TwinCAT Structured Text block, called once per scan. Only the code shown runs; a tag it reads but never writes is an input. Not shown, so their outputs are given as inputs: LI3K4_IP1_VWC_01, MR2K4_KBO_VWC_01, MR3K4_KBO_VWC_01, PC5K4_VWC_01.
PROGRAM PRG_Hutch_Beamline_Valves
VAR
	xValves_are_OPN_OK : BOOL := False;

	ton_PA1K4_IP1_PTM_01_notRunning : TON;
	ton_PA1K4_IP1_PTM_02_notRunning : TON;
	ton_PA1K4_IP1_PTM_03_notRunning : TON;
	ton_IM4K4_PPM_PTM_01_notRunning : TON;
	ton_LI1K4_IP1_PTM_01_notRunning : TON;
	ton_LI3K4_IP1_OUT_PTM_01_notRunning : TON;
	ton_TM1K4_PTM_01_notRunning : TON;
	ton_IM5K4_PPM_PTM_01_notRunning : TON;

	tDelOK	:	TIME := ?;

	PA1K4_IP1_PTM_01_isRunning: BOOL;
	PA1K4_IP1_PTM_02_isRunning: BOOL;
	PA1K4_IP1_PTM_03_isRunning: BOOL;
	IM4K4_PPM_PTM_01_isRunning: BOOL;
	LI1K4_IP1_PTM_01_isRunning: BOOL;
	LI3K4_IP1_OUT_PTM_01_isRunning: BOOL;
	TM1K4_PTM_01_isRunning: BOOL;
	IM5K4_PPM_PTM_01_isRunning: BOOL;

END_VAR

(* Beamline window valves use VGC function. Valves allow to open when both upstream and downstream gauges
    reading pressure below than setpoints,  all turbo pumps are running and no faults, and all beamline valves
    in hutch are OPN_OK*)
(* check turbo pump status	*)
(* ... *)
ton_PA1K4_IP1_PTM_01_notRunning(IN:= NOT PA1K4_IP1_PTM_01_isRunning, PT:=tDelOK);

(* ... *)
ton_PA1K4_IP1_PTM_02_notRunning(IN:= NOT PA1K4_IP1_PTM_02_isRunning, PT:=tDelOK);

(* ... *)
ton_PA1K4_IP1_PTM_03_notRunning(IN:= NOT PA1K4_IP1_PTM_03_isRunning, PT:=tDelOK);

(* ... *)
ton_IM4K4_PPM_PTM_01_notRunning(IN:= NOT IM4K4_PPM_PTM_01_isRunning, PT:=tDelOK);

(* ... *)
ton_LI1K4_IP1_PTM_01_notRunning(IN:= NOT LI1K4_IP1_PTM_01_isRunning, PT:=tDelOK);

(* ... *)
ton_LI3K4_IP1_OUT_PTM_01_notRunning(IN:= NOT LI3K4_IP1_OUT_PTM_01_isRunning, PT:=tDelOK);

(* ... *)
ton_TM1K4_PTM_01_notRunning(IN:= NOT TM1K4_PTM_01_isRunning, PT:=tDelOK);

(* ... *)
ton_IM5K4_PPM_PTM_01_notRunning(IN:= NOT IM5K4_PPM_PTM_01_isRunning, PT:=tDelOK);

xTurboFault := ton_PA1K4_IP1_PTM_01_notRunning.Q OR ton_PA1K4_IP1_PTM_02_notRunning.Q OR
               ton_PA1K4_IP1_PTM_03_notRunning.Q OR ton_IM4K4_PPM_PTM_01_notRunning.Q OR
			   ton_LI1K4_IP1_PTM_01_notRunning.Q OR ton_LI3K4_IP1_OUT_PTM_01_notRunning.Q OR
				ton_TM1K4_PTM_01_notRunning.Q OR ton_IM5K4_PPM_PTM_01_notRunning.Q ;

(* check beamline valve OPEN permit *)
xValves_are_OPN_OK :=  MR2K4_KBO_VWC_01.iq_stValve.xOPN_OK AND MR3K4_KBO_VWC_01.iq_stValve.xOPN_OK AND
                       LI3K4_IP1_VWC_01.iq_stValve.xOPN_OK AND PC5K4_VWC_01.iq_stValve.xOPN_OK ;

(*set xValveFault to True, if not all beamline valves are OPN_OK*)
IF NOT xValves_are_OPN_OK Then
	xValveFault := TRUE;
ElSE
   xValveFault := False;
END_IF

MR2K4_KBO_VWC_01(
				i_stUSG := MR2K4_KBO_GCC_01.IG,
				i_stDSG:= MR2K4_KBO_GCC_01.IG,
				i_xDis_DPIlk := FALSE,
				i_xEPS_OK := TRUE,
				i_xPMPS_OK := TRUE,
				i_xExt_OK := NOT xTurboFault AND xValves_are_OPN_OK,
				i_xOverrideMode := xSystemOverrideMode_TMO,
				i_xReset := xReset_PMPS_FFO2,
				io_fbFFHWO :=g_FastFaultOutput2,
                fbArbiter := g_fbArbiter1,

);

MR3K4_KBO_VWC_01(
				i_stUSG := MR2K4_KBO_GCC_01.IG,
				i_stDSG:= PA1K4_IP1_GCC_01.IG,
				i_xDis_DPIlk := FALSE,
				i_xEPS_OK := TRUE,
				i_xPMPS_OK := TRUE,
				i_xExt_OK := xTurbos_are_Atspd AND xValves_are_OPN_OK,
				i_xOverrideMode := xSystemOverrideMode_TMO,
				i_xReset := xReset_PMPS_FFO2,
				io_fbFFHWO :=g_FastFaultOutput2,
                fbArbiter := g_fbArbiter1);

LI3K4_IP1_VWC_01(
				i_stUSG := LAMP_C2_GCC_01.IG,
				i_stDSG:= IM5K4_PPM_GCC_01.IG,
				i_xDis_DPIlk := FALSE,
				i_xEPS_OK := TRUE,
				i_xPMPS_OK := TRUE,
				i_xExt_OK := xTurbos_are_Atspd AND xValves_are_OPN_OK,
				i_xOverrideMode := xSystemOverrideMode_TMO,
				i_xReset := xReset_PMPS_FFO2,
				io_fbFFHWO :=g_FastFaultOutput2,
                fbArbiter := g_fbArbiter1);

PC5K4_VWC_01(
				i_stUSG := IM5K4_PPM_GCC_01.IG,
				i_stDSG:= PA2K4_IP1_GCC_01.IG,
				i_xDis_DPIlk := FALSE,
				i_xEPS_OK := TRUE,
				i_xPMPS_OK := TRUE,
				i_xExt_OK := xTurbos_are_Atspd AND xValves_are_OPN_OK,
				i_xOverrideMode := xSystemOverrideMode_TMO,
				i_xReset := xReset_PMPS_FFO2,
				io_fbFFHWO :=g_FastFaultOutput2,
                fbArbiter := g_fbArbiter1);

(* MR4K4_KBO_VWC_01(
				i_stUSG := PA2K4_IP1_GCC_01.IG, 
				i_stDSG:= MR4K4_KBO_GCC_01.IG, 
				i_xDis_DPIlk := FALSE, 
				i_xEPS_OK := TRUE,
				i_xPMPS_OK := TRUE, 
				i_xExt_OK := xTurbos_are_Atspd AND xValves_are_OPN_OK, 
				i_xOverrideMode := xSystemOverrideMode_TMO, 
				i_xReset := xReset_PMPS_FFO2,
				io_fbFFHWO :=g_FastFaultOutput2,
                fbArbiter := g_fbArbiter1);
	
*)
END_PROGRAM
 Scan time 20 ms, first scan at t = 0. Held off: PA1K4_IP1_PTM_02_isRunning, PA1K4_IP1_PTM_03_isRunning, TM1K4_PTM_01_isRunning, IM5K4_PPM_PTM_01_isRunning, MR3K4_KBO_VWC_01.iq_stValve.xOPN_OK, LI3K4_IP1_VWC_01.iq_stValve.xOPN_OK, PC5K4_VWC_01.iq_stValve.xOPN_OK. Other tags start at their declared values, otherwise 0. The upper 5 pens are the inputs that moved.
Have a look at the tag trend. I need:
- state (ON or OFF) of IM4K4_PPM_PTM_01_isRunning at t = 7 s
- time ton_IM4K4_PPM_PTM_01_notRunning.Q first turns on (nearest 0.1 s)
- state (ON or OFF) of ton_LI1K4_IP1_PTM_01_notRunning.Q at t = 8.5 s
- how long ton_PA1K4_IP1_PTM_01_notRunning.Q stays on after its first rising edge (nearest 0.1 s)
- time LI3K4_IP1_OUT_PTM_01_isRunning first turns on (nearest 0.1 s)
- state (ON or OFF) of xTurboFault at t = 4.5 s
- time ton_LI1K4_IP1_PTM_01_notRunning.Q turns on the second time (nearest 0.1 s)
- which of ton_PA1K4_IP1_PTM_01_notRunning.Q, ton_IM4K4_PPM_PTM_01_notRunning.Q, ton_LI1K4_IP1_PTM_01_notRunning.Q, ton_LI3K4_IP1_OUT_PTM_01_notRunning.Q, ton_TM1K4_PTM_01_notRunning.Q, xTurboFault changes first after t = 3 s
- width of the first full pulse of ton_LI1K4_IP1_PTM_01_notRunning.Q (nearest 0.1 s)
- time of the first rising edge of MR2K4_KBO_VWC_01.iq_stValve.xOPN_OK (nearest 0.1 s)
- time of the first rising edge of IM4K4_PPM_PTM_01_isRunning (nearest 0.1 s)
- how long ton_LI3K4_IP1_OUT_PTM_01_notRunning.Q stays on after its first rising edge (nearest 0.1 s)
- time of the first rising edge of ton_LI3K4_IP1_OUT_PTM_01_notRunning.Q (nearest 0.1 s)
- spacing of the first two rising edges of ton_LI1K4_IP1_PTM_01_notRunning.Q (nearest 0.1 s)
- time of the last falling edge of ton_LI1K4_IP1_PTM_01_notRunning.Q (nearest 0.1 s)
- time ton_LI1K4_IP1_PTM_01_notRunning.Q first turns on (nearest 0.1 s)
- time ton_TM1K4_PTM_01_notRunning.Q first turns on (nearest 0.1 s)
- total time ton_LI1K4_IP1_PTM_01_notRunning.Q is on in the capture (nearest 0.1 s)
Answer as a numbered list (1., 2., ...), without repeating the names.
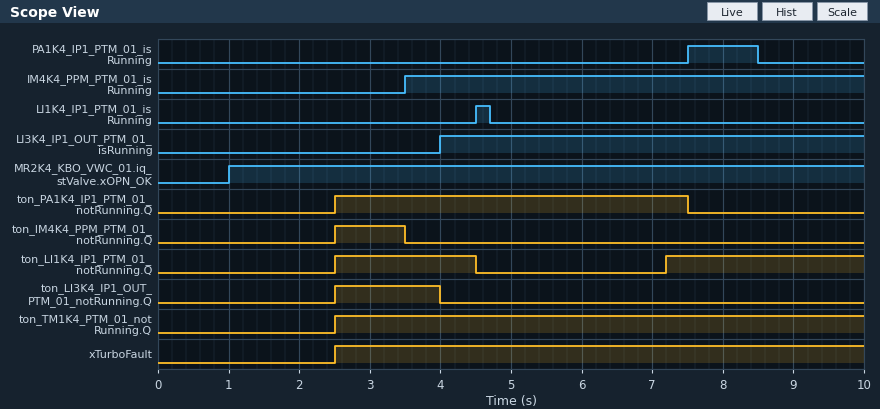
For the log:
1. ON
2. 2.5 s
3. ON
4. 5.0 s
5. 4.0 s
6. ON
7. 7.2 s
8. ton_IM4K4_PPM_PTM_01_notRunning.Q
9. 2.0 s
10. 1.0 s
11. 3.5 s
12. 1.5 s
13. 2.5 s
14. 4.7 s
15. 4.5 s
16. 2.5 s
17. 2.5 s
18. 4.8 s
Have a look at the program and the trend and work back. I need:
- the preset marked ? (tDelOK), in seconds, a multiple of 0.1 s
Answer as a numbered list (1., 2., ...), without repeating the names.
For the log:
1. 2.5 s
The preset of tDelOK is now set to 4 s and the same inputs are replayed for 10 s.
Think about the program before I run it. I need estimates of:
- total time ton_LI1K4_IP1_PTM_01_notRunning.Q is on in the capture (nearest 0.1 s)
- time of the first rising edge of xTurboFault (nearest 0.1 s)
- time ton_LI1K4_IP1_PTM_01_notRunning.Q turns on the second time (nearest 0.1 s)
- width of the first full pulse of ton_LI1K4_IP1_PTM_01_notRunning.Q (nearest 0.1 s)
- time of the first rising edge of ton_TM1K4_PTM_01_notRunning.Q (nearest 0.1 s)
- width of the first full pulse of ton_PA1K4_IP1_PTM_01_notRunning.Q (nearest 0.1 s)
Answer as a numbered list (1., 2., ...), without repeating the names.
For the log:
1. 1.8 s
2. 4.0 s
3. 8.7 s
4. 0.5 s
5. 4.0 s
6. 3.5 s
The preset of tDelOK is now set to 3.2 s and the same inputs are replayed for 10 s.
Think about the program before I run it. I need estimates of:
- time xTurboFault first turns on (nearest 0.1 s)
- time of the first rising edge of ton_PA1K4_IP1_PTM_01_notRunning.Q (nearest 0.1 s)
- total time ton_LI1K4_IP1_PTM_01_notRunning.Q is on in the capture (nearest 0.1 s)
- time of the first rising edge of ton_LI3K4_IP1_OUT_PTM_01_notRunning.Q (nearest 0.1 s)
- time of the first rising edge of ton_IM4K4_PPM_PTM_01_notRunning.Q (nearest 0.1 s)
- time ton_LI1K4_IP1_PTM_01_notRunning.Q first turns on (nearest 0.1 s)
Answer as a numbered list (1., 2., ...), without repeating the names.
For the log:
1. 3.2 s
2. 3.2 s
3. 3.4 s
4. 3.2 s
5. 3.2 s
6. 3.2 s
